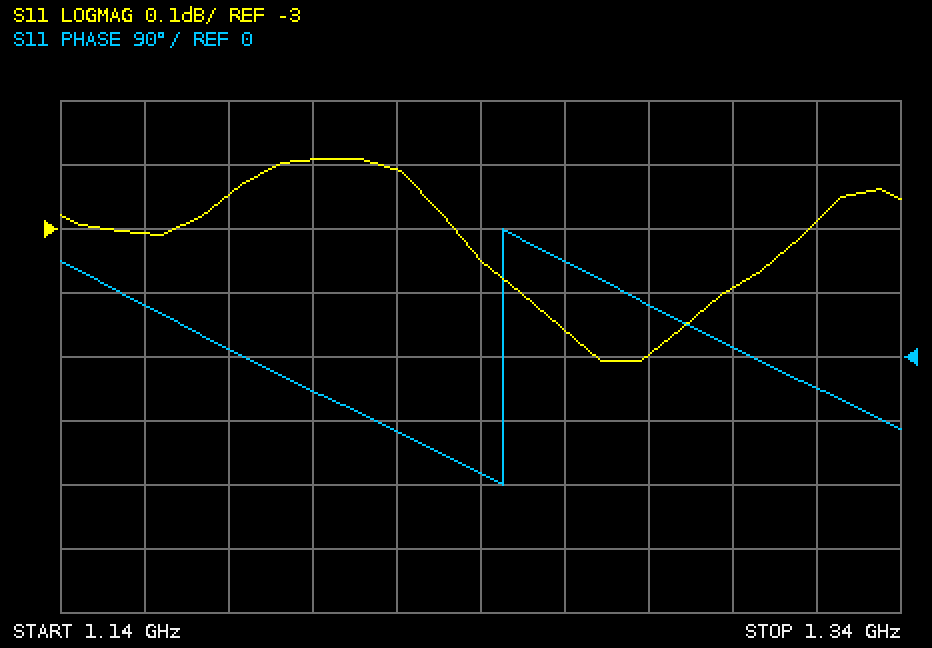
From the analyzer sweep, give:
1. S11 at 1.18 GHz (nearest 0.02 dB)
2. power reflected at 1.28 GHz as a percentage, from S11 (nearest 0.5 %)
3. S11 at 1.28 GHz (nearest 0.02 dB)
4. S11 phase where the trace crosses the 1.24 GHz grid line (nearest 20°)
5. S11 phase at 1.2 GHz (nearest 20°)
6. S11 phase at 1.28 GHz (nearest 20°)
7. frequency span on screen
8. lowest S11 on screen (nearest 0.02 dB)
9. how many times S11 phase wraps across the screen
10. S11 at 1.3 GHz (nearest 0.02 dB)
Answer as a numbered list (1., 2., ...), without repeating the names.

1. -2.94 dB
2. 48.0 %
3. -3.20 dB
4. -160°
5. -40°
6. 80°
7. 200 MHz
8. -3.20 dB
9. 1
10. -3.10 dB
